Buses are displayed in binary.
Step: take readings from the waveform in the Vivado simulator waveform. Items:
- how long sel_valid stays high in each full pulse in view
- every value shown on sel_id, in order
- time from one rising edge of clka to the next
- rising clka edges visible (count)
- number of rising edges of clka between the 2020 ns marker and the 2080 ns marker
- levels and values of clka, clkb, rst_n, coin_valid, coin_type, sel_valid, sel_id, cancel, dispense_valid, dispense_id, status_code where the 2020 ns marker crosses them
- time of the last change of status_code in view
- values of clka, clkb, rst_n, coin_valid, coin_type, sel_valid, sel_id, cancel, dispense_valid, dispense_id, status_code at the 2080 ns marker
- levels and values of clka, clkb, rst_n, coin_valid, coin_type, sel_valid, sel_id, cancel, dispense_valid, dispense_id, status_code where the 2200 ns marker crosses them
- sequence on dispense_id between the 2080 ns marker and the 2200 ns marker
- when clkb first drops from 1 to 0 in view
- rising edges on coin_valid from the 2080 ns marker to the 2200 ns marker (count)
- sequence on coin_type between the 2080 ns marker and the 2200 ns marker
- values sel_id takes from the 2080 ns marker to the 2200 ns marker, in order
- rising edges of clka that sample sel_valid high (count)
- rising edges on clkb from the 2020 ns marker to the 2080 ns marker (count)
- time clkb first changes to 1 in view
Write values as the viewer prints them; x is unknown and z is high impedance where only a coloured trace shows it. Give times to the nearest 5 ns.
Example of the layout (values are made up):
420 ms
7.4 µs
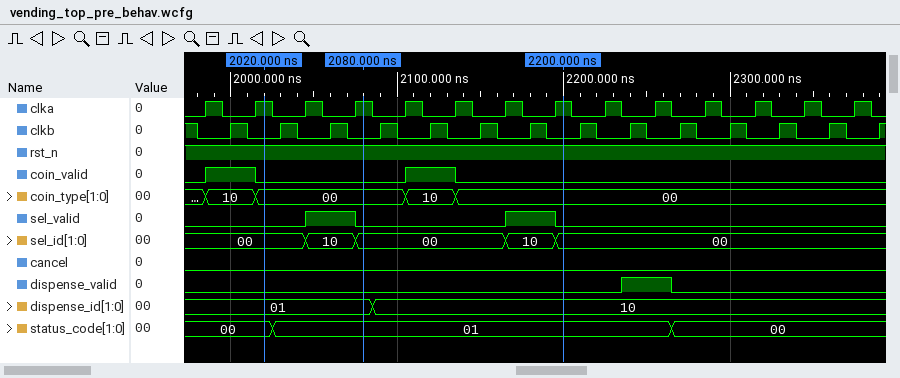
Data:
30 ns, 30 ns
00, 10, 00, 10, 00
30 ns
14
2
clka=1, clkb=0, rst_n=1, coin_valid=0, coin_type=00, sel_valid=0, sel_id=00, cancel=0, dispense_valid=0, dispense_id=01, status_code=00
2265 ns
clka=1, clkb=0, rst_n=1, coin_valid=0, coin_type=00, sel_valid=0, sel_id=00, cancel=0, dispense_valid=0, dispense_id=01, status_code=01
clka=1, clkb=0, rst_n=1, coin_valid=0, coin_type=00, sel_valid=0, sel_id=00, cancel=0, dispense_valid=0, dispense_id=10, status_code=01
01, 10
1980 ns
1
00, 10, 00
00, 10, 00
2
2
2000 ns
